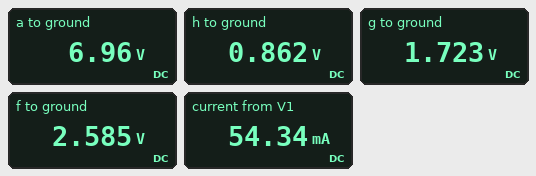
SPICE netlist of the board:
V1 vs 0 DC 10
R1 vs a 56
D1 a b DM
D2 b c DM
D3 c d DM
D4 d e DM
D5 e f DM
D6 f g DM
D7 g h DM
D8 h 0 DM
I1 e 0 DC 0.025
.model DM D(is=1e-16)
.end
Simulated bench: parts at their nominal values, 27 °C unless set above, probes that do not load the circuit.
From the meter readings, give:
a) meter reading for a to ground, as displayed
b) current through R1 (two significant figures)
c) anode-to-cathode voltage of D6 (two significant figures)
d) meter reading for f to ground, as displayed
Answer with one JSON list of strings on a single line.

["6.96 V", "54 mA", "860 mV", "2.585 V"]
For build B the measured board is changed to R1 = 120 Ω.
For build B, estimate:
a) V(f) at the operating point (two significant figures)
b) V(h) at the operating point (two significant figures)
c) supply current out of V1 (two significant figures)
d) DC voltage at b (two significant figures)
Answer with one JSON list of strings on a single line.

["2.4 V", "800 mV", "28 mA", "5.8 V"]
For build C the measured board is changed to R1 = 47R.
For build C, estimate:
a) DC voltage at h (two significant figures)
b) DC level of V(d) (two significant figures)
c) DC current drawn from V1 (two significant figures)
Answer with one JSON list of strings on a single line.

["870 mV", "4.4 V", "64 mA"]
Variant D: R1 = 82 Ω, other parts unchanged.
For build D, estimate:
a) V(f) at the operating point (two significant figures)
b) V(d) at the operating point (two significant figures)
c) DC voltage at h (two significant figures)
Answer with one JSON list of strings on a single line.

["2.5 V", "4.2 V", "840 mV"]
